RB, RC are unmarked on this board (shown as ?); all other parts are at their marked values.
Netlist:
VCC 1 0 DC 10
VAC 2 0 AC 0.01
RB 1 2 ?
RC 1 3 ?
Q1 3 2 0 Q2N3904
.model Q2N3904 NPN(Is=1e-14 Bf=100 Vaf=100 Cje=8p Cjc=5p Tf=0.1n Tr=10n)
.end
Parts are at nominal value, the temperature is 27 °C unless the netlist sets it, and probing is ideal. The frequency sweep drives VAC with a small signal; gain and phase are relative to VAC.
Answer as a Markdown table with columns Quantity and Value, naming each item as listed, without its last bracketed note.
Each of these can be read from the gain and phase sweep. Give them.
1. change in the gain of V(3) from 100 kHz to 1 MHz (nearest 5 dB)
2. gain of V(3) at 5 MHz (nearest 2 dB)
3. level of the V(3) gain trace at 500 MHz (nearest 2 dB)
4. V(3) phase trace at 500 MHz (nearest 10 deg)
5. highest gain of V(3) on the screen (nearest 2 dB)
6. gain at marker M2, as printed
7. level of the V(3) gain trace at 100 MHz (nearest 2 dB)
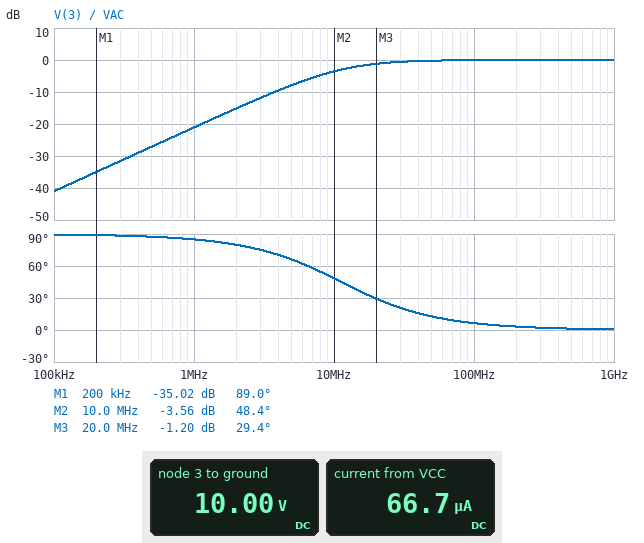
| Quantity | Value |
|---|---|
| change in the gain of V(3) from 100 kHz to 1 MHz | 20 dB |
| gain of V(3) at 5 MHz | -8 dB |
| level of the V(3) gain trace at 500 MHz | 0 dB |
| V(3) phase trace at 500 MHz | 0 deg |
| highest gain of V(3) on the screen | 0 dB |
| gain at marker M2, as printed | -3.56 dB |
| level of the V(3) gain trace at 100 MHz | 0 dB |
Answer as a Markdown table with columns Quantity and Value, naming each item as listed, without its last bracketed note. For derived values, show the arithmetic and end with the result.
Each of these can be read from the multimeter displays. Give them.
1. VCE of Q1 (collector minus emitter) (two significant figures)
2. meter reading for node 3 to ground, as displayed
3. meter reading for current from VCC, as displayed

| Quantity | Value |
|---|---|
| VCE of Q1 (collector minus emitter) | 10 V = 10 V |
| meter reading for node 3 to ground, as displayed | 10.00 V |
| meter reading for current from VCC, as displayed | 66.7 µA |
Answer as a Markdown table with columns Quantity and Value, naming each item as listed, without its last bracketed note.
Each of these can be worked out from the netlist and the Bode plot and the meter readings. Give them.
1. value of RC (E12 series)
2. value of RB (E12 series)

| Quantity | Value |
|---|---|
| value of RC | 6.8 kΩ |
| value of RB | 150 kΩ |
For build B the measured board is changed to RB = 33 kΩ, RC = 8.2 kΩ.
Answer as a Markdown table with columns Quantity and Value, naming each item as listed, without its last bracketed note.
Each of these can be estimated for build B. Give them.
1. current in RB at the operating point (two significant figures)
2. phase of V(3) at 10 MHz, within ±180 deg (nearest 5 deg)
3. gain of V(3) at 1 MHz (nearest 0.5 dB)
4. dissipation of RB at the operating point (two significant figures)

| Quantity | Value |
|---|---|
| current in RB at the operating point | 300 µA |
| phase of V(3) at 10 MHz, within ±180 deg | 45 deg |
| gain of V(3) at 1 MHz | -19.5 dB |
| dissipation of RB at the operating point | 3.0 mW |
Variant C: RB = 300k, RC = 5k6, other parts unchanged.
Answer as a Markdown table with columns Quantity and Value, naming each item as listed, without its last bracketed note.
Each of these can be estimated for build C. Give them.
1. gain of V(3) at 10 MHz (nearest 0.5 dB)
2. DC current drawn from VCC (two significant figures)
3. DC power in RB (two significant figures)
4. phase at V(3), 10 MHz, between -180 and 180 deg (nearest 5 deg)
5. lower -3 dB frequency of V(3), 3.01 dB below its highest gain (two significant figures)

| Quantity | Value |
|---|---|
| gain of V(3) at 10 MHz | -4.5 dB |
| DC current drawn from VCC | 33 µA |
| DC power in RB | 330 µW |
| phase at V(3), 10 MHz, between -180 and 180 deg | 55 deg |
| lower -3 dB frequency of V(3), 3.01 dB below its highest gain | 14 MHz |
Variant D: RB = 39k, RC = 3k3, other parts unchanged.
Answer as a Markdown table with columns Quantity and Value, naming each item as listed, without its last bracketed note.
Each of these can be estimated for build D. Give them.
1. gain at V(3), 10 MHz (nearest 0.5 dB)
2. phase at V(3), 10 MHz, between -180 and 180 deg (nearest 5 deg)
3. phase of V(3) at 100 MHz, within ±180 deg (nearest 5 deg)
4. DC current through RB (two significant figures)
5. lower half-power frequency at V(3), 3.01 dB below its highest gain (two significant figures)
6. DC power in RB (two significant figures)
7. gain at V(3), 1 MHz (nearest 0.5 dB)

| Quantity | Value |
|---|---|
| gain at V(3), 10 MHz | -8.0 dB |
| phase at V(3), 10 MHz, between -180 and 180 deg | 65 deg |
| phase of V(3) at 100 MHz, within ±180 deg | 15 deg |
| DC current through RB | 260 µA |
| lower half-power frequency at V(3), 3.01 dB below its highest gain | 23 MHz |
| DC power in RB | 2.6 mW |
| gain at V(3), 1 MHz | -27.5 dB |
